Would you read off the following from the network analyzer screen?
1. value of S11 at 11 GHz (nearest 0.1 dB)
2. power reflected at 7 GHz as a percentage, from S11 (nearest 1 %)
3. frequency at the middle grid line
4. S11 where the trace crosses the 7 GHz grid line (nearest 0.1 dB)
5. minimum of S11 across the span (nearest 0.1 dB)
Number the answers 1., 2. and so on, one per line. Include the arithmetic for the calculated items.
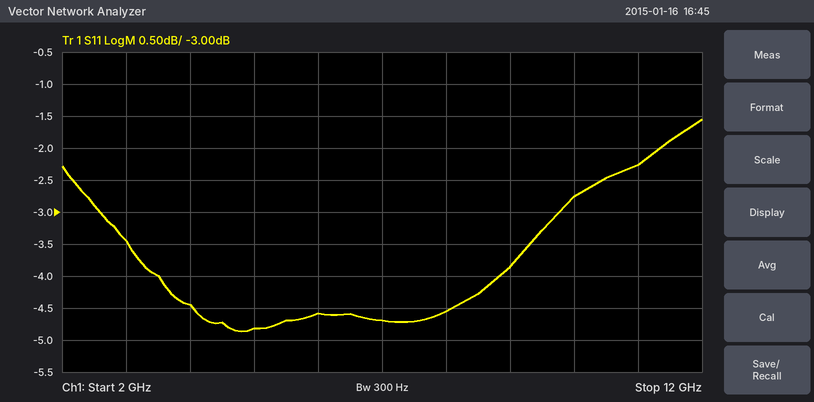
1. -2.3 dB
2. 10^(-4.7/10) ≈ 34 %
3. 7 GHz
4. -4.7 dB
5. -4.9 dB
